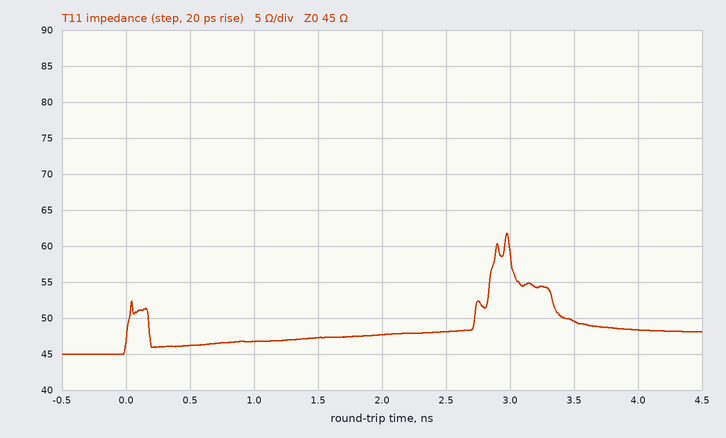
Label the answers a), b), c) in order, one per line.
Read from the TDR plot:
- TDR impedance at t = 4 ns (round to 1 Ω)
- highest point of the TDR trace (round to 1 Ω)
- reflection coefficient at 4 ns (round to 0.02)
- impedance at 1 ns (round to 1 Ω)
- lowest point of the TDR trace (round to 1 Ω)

a) 48 Ω
b) 62 Ω
c) +0.04
d) 47 Ω
e) 45 Ω
